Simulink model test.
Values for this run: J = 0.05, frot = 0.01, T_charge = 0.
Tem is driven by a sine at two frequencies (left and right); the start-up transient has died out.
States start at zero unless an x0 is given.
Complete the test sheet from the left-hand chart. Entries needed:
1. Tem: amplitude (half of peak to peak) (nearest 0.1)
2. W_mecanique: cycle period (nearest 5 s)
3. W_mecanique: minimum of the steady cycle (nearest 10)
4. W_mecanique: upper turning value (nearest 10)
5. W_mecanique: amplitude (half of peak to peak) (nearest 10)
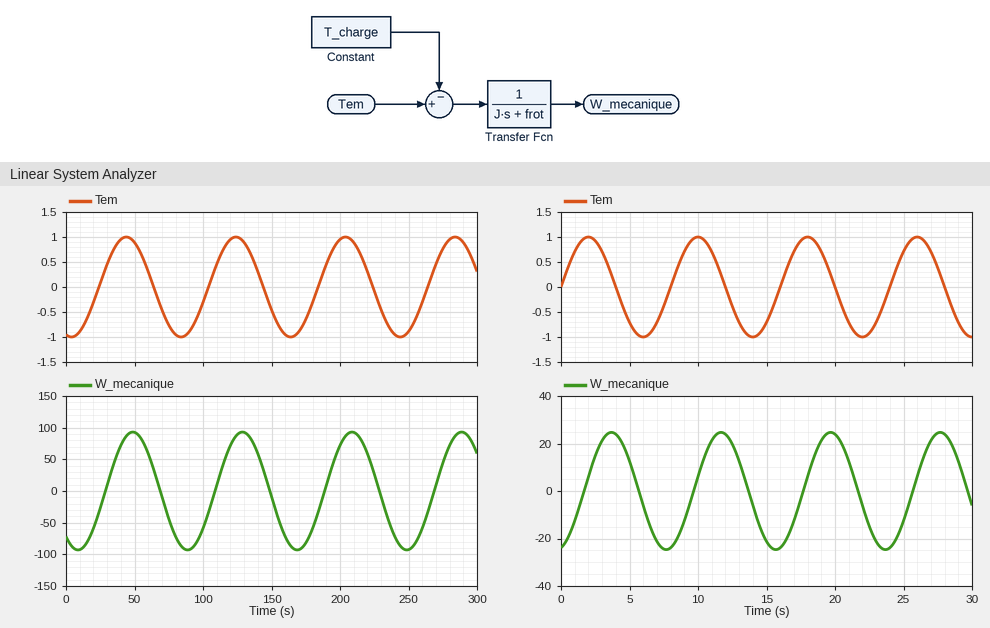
1.0
80 s
-90
90
90
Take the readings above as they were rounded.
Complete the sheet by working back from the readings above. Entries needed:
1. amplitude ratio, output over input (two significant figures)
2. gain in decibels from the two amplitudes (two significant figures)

90
39 dB
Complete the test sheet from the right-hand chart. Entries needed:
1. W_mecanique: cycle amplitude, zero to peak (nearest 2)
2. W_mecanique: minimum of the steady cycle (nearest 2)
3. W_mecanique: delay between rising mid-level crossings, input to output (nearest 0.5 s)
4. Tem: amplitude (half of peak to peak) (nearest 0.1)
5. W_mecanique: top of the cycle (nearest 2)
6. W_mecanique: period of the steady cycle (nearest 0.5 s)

24
-24
1.5 s
1.0
24
8.0 s
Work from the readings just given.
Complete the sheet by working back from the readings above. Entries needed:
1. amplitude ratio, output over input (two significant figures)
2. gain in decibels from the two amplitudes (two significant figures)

24
28 dB
